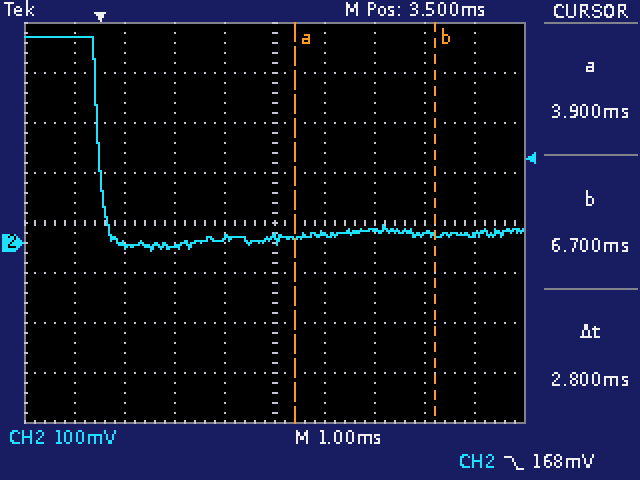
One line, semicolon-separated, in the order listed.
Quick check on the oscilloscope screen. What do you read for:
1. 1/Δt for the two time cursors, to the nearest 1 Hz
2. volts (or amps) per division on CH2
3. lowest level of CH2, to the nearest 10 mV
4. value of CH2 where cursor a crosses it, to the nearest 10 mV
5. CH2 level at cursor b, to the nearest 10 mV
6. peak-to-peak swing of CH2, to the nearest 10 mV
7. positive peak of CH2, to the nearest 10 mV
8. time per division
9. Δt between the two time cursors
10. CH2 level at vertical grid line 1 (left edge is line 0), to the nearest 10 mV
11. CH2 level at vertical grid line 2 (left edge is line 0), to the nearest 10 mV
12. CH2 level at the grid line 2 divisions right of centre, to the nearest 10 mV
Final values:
357 Hz; 100 mV; -20 mV; 10 mV; 20 mV; 430 mV; 410 mV; 1 ms; 2.8 ms; 410 mV; 0 mV; 30 mV
